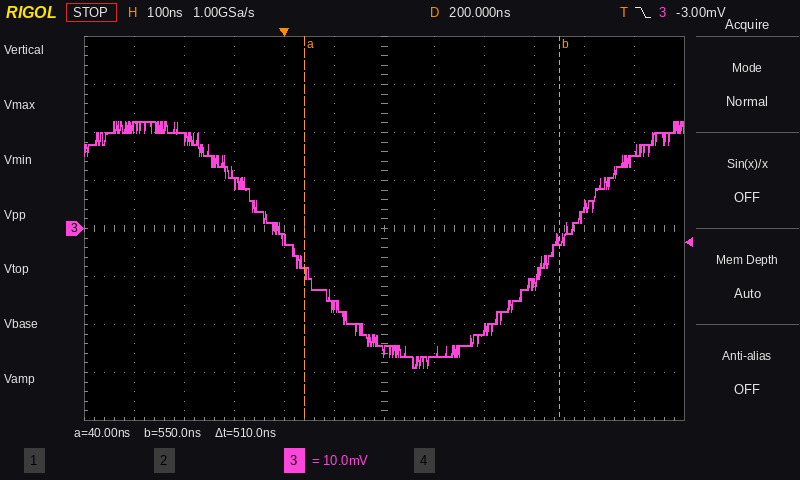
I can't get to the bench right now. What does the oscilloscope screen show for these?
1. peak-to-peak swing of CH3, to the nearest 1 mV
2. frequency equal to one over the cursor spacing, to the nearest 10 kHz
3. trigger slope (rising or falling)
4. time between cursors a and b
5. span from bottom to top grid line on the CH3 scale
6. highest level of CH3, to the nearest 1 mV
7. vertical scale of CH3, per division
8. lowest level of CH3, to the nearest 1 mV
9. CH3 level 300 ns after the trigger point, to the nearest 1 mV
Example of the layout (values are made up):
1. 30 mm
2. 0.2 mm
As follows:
1. 51 mV
2. 1.96 MHz
3. falling
4. 510 ns
5. 80 mV
6. 22 mV
7. 10 mV
8. -29 mV
9. -26 mV
